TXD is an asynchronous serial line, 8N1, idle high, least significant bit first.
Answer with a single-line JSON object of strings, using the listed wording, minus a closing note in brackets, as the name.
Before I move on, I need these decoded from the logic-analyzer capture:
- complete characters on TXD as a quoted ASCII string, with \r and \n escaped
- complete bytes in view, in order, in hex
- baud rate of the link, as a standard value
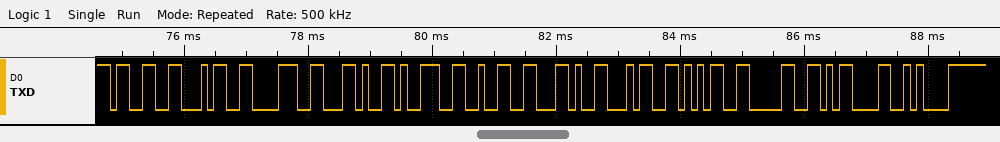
{"complete characters on TXD as a quoted ASCII string, with \\r and \\n escaped": "\"348,92,450\\r\\n\"", "complete bytes in view, in order, in hex": "0x33 0x34 0x38 0x2C 0x39 0x32 0x2C 0x34 0x35 0x30 0x0D 0x0A", "baud rate of the link, as a standard value": "9600 baud"}
